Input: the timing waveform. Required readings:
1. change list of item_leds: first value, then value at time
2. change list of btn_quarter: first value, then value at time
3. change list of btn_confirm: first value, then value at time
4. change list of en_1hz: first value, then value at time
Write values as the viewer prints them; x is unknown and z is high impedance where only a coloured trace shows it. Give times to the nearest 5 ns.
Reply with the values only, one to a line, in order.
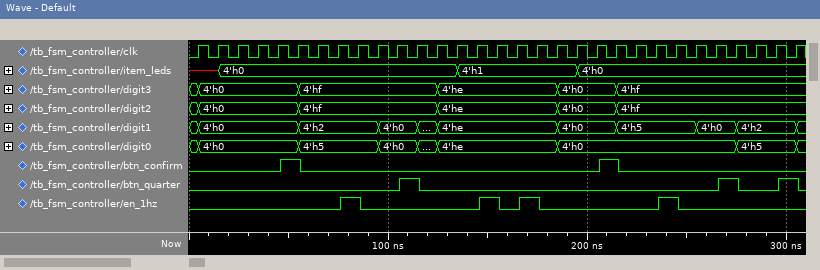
x, 4'h0 at 15 ns, 4'h1 at 135 ns, 4'h0 at 195 ns
0, 1 at 105 ns, 0 at 115 ns, 1 at 265 ns, 0 at 275 ns, 1 at 295 ns, 0 at 305 ns
0, 1 at 45 ns, 0 at 55 ns, 1 at 205 ns, 0 at 215 ns
0, 1 at 75 ns, 0 at 85 ns, 1 at 145 ns, 0 at 155 ns, 1 at 165 ns, 0 at 175 ns, 1 at 235 ns, 0 at 245 ns
